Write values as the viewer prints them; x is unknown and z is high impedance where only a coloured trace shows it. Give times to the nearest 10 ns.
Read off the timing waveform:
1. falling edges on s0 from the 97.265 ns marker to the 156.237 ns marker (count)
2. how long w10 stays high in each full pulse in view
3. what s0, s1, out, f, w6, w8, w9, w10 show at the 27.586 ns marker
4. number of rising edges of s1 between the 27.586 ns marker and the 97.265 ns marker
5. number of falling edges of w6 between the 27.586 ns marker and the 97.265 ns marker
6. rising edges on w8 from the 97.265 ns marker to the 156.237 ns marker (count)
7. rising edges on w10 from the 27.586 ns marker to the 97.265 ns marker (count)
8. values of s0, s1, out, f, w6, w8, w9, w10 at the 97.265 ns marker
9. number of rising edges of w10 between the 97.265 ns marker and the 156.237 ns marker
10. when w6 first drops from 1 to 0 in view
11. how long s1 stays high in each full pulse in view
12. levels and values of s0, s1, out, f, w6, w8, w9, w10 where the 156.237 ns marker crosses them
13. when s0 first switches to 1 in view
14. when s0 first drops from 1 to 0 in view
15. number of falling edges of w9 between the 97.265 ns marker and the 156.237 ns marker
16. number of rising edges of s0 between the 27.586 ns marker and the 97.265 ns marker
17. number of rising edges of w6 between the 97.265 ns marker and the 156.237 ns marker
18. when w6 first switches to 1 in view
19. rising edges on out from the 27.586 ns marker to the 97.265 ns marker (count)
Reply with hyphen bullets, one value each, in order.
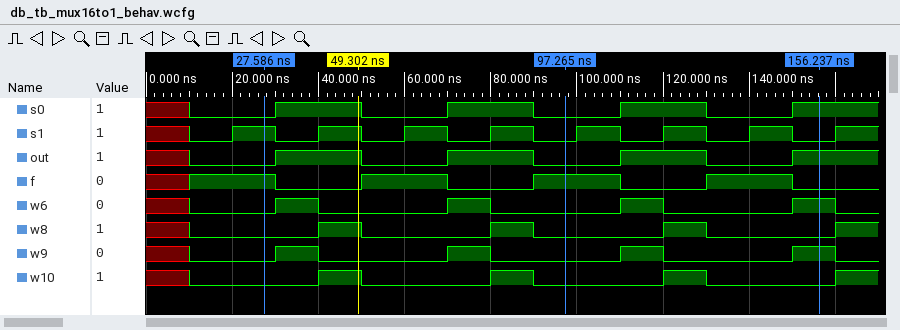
- 1
- 10 ns, 10 ns, 10 ns
- s0=0, s1=1, out=0, f=1, w6=0, w8=0, w9=0, w10=0
- 3
- 2
- 1
- 2
- s0=0, s1=0, out=0, f=1, w6=0, w8=0, w9=0, w10=0
- 1
- 40 ns
- 10 ns, 10 ns, 10 ns, 10 ns, 10 ns, 10 ns, 10 ns
- s0=1, s1=0, out=1, f=0, w6=1, w8=0, w9=1, w10=0
- 30 ns
- 50 ns
- 1
- 2
- 2
- 30 ns
- 2
